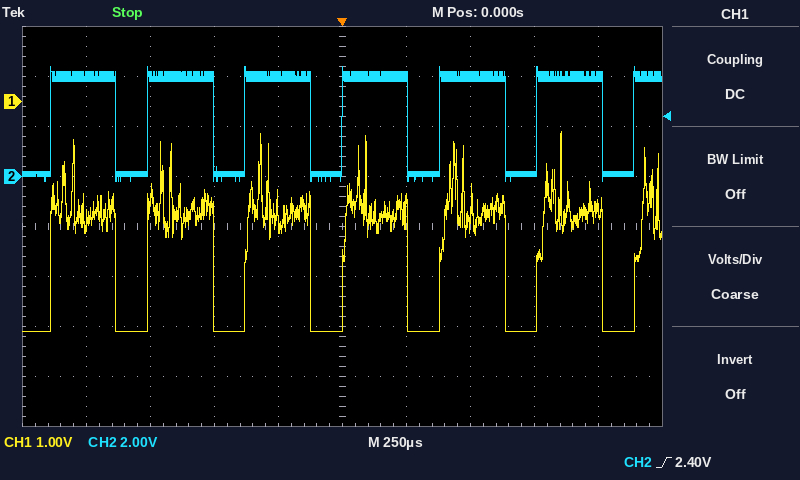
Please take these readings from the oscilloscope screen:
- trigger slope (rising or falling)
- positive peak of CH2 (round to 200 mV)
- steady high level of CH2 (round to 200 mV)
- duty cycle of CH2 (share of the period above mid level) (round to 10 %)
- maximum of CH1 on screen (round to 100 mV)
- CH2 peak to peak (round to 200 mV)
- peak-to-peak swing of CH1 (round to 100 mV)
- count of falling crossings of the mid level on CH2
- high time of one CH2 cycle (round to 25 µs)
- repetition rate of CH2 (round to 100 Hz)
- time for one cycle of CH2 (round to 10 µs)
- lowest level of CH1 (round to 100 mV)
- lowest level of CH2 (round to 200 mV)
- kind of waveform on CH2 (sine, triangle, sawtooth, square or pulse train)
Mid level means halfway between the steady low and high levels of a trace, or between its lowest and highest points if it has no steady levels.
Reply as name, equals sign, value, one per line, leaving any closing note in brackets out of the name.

trigger slope = rising
positive peak of CH2 = 4.4 V
steady high level of CH2 = 4.0 V
duty cycle of CH2 (share of the period above mid level) = 70 %
maximum of CH1 on screen = -600 mV
CH2 peak to peak = 4.6 V
peak-to-peak swing of CH1 = 4.0 V
count of falling crossings of the mid level on CH2 = 6
high time of one CH2 cycle = 250 µs
repetition rate of CH2 = 2.6 kHz
time for one cycle of CH2 = 380 µs
lowest level of CH1 = -4.6 V
lowest level of CH2 = -200 mV
kind of waveform on CH2 = pulse train
